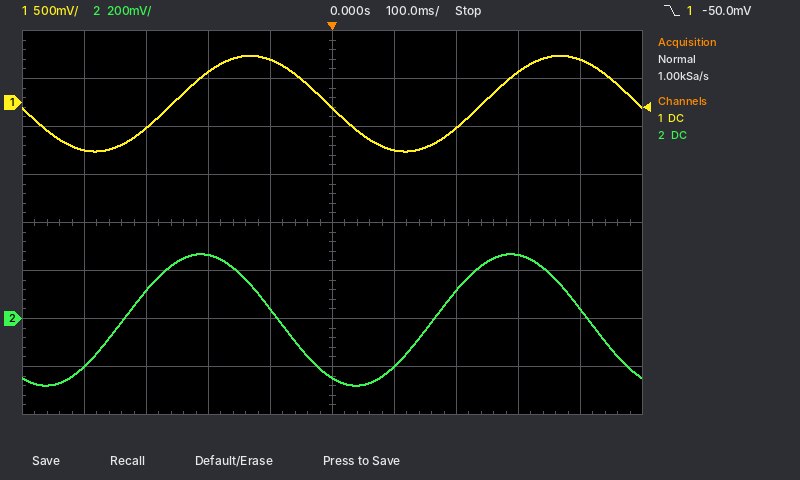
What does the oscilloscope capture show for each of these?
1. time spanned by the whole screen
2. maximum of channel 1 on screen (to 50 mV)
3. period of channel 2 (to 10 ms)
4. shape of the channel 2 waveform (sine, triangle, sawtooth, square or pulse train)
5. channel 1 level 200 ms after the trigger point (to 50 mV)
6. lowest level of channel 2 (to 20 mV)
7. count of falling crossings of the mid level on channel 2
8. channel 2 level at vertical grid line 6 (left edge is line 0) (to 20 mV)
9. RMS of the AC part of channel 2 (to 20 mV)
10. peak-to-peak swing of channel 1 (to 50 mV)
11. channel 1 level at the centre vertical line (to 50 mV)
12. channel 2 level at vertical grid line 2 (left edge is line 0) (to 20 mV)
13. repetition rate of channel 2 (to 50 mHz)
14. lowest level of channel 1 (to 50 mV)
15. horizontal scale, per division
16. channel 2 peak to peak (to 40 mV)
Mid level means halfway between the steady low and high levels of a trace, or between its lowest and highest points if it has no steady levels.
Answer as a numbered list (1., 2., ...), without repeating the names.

1. 1 s
2. 500 mV
3. 500 ms
4. sine
5. -250 mV
6. -280 mV
7. 2
8. -200 mV
9. 200 mV
10. 1.00 V
11. -50 mV
12. 120 mV
13. 2.00 Hz
14. -500 mV
15. 100 ms
16. 560 mV
